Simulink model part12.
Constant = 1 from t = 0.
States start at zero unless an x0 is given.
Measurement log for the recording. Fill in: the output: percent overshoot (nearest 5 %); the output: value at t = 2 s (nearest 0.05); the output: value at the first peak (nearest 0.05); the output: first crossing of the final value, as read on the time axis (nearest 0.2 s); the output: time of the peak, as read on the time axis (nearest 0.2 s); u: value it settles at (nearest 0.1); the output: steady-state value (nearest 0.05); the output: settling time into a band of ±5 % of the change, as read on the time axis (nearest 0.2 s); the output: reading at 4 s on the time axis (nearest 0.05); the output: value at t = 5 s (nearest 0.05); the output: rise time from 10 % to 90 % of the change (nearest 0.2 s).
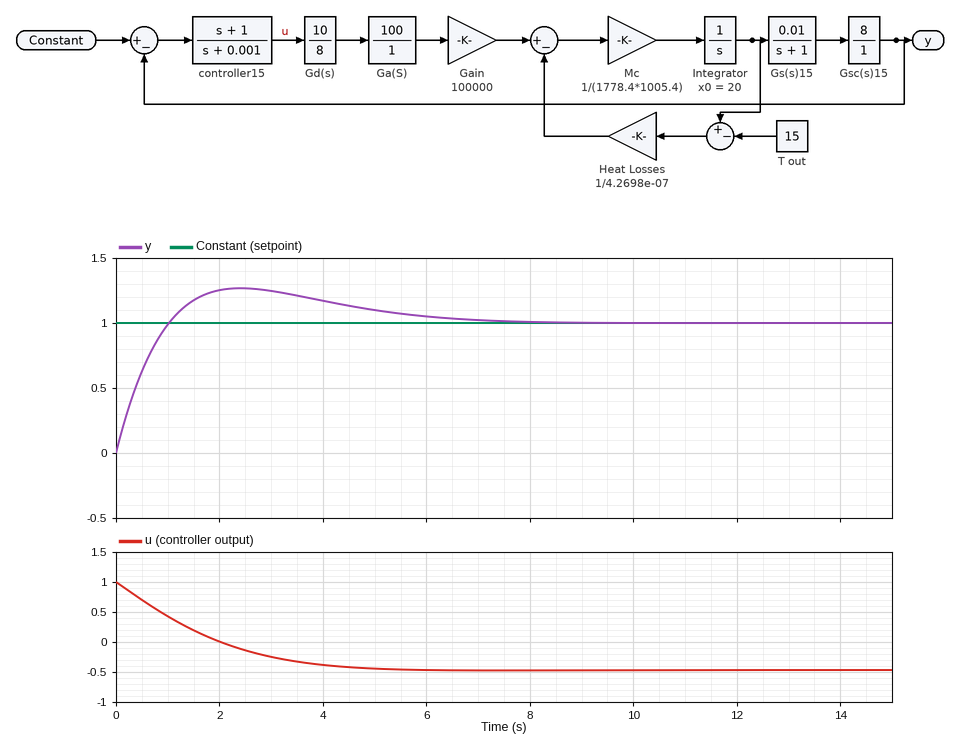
25 %
1.25
1.25
1.0 s
2.4 s
-0.5
1.00
6.0 s
1.15
1.10
0.8 s
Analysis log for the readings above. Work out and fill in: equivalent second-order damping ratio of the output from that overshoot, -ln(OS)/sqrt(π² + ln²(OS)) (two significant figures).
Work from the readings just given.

0.40
